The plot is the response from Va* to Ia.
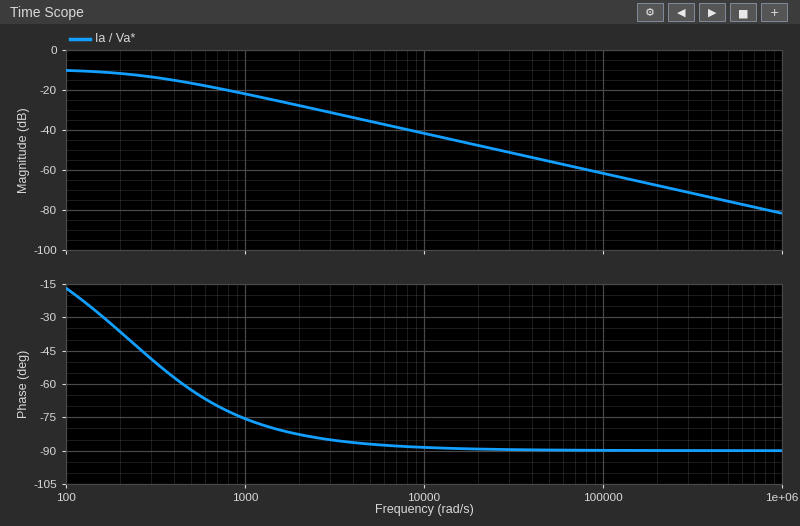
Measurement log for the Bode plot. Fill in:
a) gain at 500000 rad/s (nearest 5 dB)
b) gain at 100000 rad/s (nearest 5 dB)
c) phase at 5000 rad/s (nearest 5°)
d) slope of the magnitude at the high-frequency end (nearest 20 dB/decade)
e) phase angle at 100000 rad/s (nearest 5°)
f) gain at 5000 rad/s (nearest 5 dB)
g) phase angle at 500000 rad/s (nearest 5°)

-75 dB
-60 dB
-85°
-20 dB/decade
-90°
-35 dB
-90°
